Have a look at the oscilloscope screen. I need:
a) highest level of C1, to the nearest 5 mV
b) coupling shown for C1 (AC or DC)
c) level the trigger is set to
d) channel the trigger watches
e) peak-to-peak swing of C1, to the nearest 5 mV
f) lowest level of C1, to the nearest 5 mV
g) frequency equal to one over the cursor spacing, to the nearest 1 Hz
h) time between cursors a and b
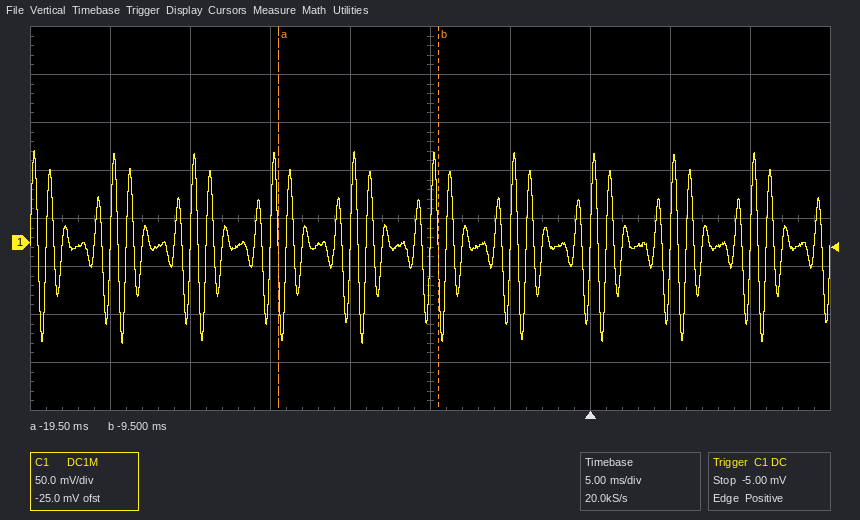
95 mV
DC
-5.00 mV
C1
200 mV
-105 mV
100 Hz
10.0 ms
